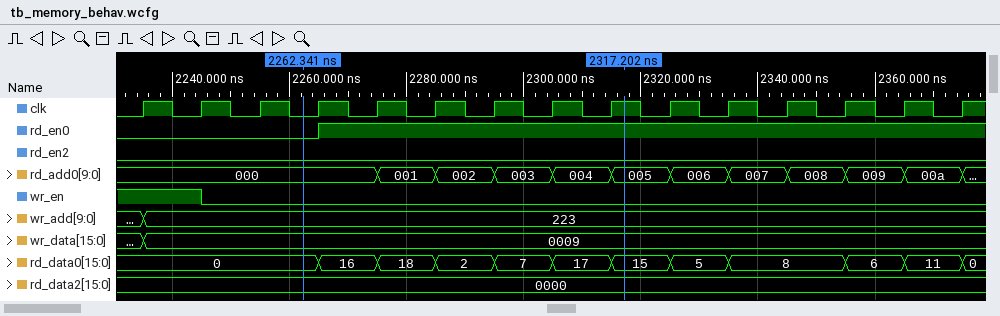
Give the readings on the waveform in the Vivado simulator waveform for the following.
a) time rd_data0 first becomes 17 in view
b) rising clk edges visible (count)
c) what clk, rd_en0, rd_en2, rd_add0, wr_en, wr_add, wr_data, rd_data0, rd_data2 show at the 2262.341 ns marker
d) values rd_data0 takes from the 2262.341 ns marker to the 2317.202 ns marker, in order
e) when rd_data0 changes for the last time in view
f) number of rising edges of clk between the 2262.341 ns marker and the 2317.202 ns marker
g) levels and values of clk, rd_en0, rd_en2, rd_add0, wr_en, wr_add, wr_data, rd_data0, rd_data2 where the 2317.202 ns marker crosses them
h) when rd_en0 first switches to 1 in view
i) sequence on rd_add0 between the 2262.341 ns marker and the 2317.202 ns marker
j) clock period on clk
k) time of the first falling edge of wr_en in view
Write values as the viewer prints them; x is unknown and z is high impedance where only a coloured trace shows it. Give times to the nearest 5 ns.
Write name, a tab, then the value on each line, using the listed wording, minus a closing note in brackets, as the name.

time rd_data0 first becomes 17 in view	2305 ns
rising clk edges visible	15
what clk, rd_en0, rd_en2, rd_add0, wr_en, wr_add, wr_data, rd_data0, rd_data2 show at the 2262.341 ns marker	clk=0, rd_en0=0, rd_en2=0, rd_add0=000, wr_en=0, wr_add=223, wr_data=0009, rd_data0=0, rd_data2=0000
values rd_data0 takes from the 2262.341 ns marker to the 2317.202 ns marker, in order	0, 16, 18, 2, 7, 17, 15
when rd_data0 changes for the last time in view	2375 ns
number of rising edges of clk between the 2262.341 ns marker and the 2317.202 ns marker	6
levels and values of clk, rd_en0, rd_en2, rd_add0, wr_en, wr_add, wr_data, rd_data0, rd_data2 where the 2317.202 ns marker crosses them	clk=1, rd_en0=1, rd_en2=0, rd_add0=005, wr_en=0, wr_add=223, wr_data=0009, rd_data0=15, rd_data2=0000
when rd_en0 first switches to 1 in view	2265 ns
sequence on rd_add0 between the 2262.341 ns marker and the 2317.202 ns marker	000, 001, 002, 003, 004, 005
clock period on clk	10 ns
time of the first falling edge of wr_en in view	2245 ns
